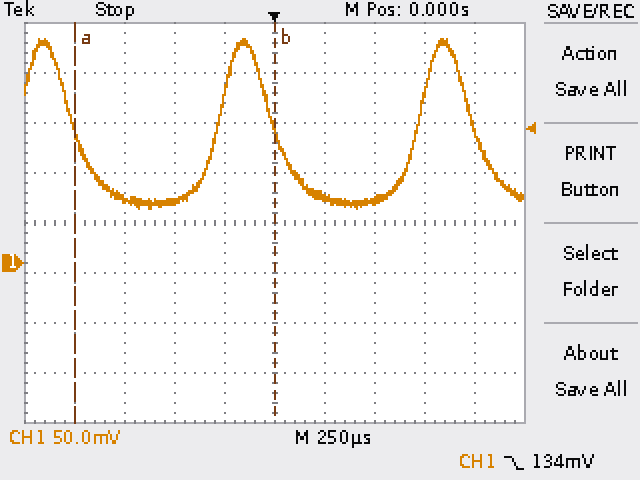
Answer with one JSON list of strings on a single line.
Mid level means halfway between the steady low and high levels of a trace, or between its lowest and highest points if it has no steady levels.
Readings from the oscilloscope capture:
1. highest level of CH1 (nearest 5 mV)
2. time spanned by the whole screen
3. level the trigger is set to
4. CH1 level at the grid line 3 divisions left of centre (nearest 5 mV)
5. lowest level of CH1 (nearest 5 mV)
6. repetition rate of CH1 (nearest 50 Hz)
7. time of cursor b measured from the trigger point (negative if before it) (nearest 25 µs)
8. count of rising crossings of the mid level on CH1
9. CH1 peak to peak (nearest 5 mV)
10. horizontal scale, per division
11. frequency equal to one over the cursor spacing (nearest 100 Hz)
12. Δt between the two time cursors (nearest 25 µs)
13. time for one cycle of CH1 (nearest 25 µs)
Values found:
["225 mV", "2.5 ms", "134 mV", "65 mV", "55 mV", "1.00 kHz", "0 µs", "2", "170 mV", "250 µs", "1.0 kHz", "1.000 ms", "1.000 ms"]
